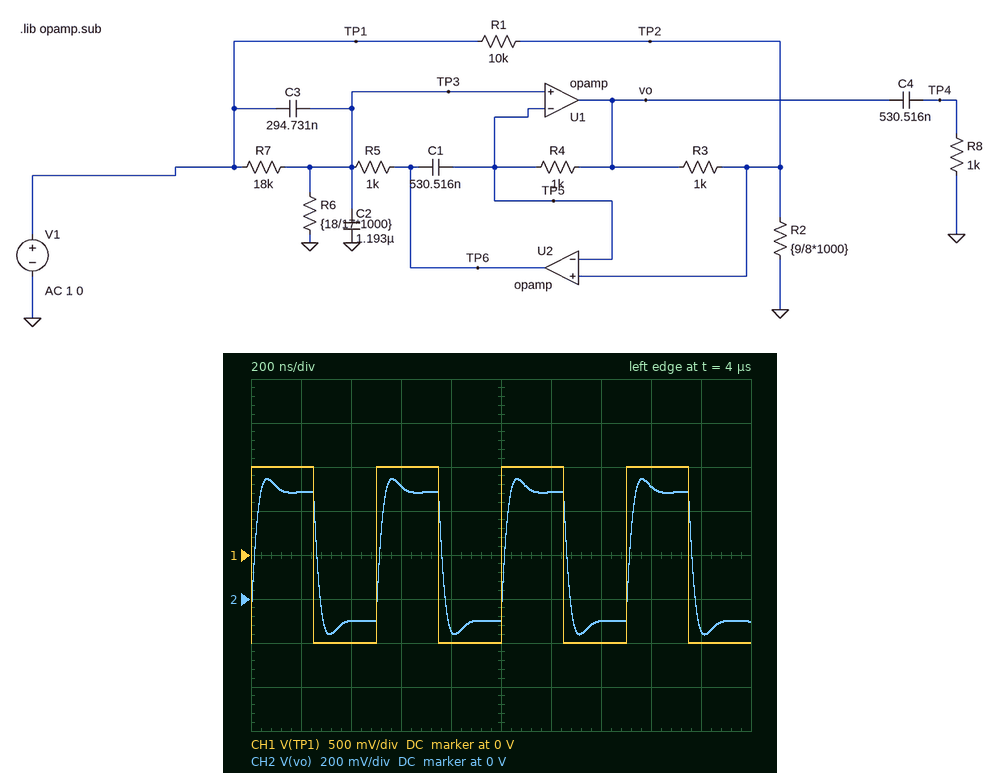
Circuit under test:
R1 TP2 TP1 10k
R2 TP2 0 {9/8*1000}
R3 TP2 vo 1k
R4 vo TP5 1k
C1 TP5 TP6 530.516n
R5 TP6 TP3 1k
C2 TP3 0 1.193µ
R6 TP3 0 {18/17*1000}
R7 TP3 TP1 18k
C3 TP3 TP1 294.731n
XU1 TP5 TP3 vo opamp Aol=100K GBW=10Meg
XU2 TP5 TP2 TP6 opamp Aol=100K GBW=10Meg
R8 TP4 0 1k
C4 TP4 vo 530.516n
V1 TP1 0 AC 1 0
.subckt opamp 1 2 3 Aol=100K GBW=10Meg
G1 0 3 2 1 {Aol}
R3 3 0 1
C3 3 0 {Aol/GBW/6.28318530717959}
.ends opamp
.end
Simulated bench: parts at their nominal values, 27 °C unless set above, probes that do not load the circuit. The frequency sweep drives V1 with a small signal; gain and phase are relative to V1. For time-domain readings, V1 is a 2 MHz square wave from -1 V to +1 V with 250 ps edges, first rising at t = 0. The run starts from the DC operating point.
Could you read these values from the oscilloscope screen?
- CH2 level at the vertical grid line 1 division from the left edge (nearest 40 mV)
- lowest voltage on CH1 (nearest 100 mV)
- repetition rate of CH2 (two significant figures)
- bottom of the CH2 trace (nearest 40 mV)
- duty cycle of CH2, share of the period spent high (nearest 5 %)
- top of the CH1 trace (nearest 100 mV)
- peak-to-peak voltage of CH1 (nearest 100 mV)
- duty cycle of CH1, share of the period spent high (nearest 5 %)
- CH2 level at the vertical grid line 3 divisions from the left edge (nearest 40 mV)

480 mV
-1.0 V
2.0 MHz
-160 mV
50 %
1.0 V
2.0 V
50 %
520 mV
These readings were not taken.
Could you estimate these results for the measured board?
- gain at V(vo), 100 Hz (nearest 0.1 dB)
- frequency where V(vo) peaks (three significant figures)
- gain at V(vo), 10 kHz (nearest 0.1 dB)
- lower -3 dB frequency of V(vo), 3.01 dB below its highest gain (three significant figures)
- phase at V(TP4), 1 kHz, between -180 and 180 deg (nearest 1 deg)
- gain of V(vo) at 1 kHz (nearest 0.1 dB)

-38.4 dB
219 Hz
-10.6 dB
166 Hz
23 deg
-10.5 dB
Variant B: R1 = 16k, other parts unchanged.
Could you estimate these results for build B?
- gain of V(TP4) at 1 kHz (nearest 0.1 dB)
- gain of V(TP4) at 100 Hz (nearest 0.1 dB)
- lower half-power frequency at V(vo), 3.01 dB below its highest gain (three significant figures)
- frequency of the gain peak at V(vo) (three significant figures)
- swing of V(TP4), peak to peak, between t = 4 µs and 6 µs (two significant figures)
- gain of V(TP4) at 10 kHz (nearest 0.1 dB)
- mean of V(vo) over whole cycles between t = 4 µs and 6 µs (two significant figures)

-10.0 dB
-34.8 dB
156 Hz
204 Hz
770 mV
-9.8 dB
260 mV
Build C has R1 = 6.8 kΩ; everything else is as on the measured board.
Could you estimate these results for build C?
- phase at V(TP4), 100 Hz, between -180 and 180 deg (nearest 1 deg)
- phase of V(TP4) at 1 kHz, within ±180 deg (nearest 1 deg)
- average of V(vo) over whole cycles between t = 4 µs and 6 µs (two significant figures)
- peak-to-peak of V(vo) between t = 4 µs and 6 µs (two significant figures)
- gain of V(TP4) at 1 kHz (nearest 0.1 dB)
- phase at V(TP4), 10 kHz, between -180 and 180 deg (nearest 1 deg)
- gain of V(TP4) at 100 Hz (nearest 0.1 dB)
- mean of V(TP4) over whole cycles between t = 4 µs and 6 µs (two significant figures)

37 deg
24 deg
110 mV
640 mV
-12.1 dB
2 deg
-31.4 dB
250 mV
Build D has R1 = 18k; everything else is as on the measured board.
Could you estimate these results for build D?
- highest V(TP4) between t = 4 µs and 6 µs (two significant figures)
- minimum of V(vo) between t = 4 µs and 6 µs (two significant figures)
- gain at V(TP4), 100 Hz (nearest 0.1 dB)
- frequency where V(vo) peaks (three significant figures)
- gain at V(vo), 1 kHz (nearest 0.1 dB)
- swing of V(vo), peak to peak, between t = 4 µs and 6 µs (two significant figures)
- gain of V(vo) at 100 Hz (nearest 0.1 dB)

710 mV
-120 mV
-33.1 dB
202 Hz
-9.5 dB
780 mV
-23.1 dB
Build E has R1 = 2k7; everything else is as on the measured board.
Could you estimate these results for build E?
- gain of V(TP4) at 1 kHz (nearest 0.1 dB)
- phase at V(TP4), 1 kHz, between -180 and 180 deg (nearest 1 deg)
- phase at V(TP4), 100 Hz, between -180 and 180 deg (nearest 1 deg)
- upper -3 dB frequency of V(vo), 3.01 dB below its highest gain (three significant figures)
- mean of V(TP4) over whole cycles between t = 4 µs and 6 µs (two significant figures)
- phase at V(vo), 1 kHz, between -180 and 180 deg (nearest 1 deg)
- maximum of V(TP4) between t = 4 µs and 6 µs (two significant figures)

-23.1 dB
45 deg
39 deg
230 Hz
75 mV
28 deg
320 mV
